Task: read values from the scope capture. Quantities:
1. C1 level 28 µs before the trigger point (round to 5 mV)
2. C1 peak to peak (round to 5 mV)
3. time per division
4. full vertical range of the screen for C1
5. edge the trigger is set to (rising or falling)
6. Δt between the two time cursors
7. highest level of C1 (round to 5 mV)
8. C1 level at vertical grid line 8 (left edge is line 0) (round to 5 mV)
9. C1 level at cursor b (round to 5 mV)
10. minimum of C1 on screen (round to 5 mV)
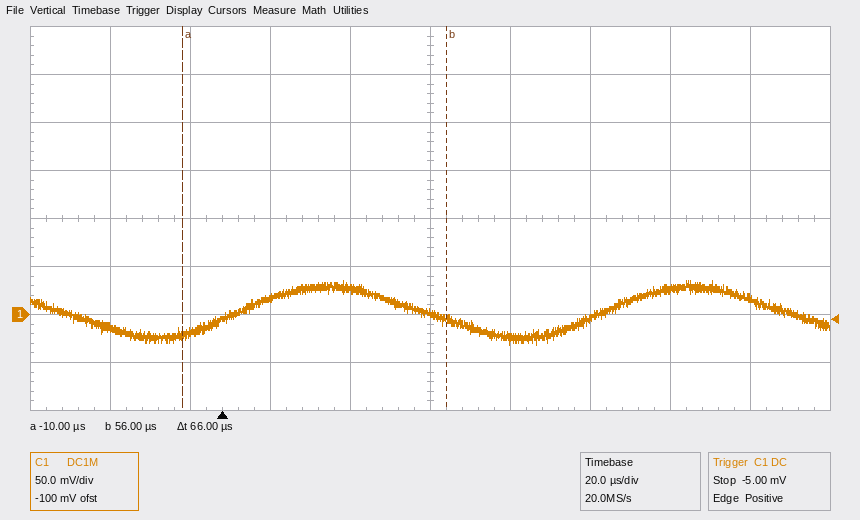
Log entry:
-15 mV
65 mV
20 µs
400 mV
rising
66 µs
35 mV
25 mV
-5 mV
-30 mV
